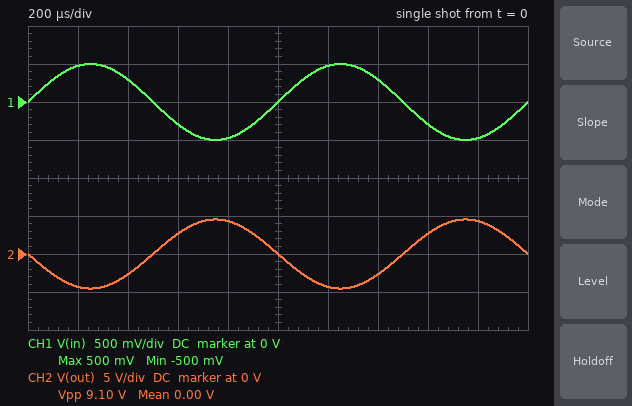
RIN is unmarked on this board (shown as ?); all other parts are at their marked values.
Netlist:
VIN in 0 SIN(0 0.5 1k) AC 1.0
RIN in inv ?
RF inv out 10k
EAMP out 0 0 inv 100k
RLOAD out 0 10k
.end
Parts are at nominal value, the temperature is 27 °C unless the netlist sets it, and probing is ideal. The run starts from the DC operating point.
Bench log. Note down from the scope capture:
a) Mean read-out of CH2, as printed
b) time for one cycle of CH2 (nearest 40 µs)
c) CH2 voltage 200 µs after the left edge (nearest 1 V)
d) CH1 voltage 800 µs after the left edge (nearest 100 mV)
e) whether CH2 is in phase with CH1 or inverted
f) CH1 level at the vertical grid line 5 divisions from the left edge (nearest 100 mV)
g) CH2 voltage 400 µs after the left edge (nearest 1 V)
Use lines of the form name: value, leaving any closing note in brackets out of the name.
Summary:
Mean read-out of CH2, as printed: 0.00 V
time for one cycle of CH2: 1.00 ms
CH2 voltage 200 µs after the left edge: -4 V
CH1 voltage 800 µs after the left edge: -500 mV
whether CH2 is in phase with CH1 or inverted: inverted
CH1 level at the vertical grid line 5 divisions from the left edge: 0 V
CH2 voltage 400 µs after the left edge: -3 V
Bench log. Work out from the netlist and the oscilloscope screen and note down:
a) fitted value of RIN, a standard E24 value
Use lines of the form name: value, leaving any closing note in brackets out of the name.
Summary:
fitted value of RIN, a standard E24 value: 1.1 kΩ
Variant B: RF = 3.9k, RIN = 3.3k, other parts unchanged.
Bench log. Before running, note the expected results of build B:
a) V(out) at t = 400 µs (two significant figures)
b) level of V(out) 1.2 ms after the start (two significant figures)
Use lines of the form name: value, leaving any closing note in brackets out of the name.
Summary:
V(out) at t = 400 µs: -350 mV
level of V(out) 1.2 ms after the start: -560 mV
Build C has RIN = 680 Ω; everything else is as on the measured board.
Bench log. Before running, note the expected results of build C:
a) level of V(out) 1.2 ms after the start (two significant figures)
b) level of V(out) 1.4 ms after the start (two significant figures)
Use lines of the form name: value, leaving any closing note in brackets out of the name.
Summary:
level of V(out) 1.2 ms after the start: -7.0 V
level of V(out) 1.4 ms after the start: -4.3 V
